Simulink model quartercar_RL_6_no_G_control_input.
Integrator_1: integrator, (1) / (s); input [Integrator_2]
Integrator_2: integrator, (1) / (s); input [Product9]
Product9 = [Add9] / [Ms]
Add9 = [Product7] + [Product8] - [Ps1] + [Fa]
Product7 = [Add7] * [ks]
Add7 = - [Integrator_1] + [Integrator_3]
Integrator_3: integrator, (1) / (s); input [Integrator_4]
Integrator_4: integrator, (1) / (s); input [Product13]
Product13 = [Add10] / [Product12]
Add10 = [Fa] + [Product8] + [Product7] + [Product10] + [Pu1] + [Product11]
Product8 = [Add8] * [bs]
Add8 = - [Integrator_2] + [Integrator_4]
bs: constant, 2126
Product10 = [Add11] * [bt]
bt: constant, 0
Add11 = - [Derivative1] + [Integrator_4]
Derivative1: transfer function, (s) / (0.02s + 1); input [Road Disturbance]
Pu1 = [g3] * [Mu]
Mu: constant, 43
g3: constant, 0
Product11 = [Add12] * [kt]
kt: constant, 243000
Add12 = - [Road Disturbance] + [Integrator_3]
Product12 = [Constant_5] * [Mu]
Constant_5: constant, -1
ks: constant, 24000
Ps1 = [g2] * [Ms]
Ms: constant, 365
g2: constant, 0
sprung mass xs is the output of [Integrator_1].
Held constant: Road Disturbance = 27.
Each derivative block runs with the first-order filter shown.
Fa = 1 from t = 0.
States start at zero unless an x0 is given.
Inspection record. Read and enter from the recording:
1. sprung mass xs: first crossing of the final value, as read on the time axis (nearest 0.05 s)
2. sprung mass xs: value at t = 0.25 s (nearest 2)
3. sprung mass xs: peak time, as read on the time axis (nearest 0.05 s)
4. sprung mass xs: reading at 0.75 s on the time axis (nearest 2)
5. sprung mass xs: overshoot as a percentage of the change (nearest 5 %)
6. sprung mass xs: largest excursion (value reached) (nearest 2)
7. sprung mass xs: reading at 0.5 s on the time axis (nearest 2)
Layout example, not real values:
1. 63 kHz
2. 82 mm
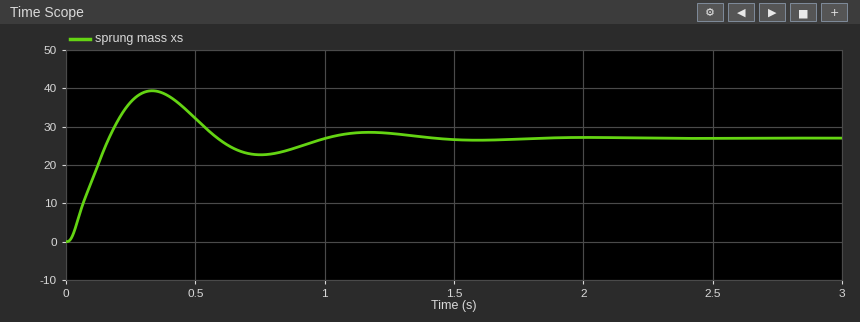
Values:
1. 0.15 s
2. 36
3. 0.35 s
4. 22
5. 45 %
6. 40
7. 32
